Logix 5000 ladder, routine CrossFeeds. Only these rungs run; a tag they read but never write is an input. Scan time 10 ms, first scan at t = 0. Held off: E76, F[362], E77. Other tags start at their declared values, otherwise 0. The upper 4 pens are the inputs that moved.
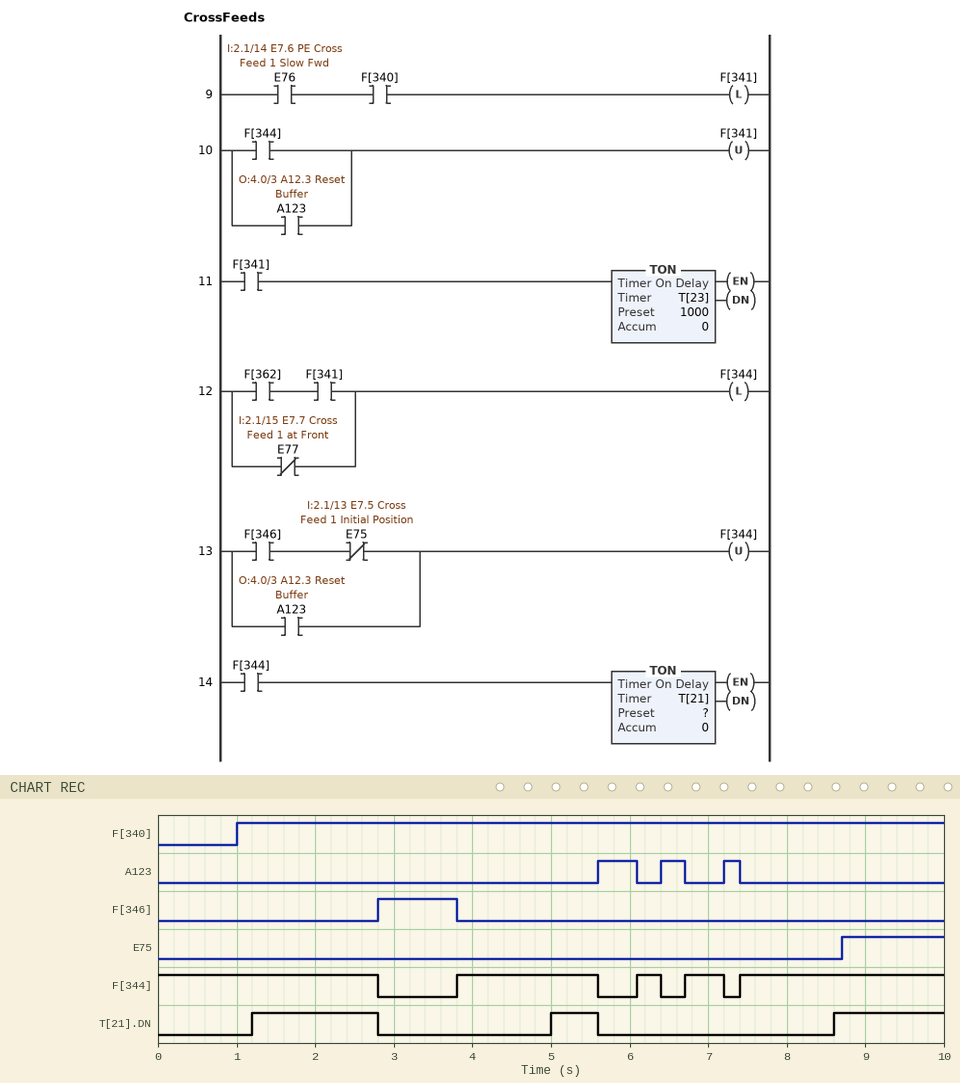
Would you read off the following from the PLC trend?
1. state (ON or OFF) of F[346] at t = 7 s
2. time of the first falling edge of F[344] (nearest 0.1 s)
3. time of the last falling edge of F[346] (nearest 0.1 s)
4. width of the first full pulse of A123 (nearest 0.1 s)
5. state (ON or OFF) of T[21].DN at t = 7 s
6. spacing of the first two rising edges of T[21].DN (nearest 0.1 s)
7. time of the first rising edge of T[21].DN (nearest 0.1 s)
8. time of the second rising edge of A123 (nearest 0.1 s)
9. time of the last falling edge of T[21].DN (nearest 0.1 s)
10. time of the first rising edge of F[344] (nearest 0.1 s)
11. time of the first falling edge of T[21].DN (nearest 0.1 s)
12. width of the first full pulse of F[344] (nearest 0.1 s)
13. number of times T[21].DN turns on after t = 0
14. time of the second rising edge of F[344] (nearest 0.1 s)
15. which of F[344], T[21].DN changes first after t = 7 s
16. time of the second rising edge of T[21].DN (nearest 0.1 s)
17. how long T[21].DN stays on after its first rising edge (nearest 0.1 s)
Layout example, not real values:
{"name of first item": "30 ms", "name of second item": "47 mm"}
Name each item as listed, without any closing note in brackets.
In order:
{"state (ON or OFF) of F[346] at t = 7 s": "OFF", "time of the first falling edge of F[344]": "2.8 s", "time of the last falling edge of F[346]": "3.8 s", "width of the first full pulse of A123": "0.5 s", "state (ON or OFF) of T[21].DN at t = 7 s": "OFF", "spacing of the first two rising edges of T[21].DN": "3.8 s", "time of the first rising edge of T[21].DN": "1.2 s", "time of the second rising edge of A123": "6.4 s", "time of the last falling edge of T[21].DN": "5.6 s", "time of the first rising edge of F[344]": "3.8 s", "time of the first falling edge of T[21].DN": "2.8 s", "width of the first full pulse of F[344]": "1.8 s", "number of times T[21].DN turns on after t = 0": "3", "time of the second rising edge of F[344]": "6.1 s", "which of F[344], T[21].DN changes first after t = 7 s": "F[344]", "time of the second rising edge of T[21].DN": "5.0 s", "how long T[21].DN stays on after its first rising edge": "1.6 s"}
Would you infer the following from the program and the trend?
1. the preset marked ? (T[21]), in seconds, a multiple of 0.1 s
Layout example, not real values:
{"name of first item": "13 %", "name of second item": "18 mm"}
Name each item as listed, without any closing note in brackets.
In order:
{"the preset marked ? (T[21]), in seconds, a multiple of 0.1 s": "1.2 s"}
